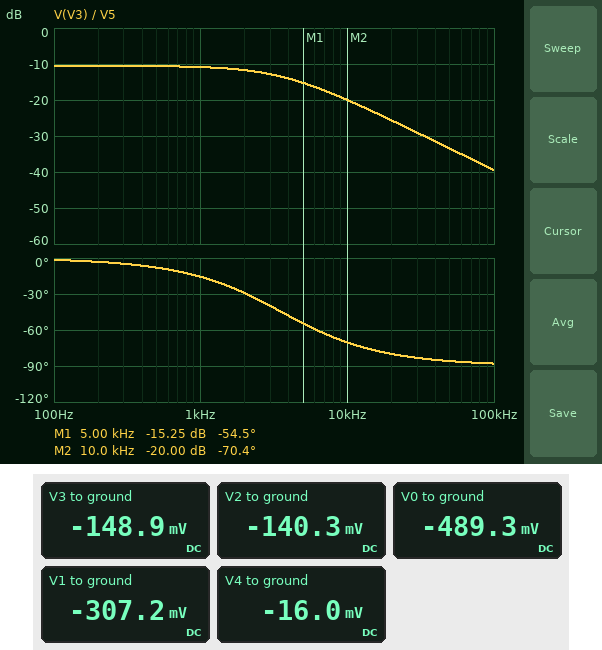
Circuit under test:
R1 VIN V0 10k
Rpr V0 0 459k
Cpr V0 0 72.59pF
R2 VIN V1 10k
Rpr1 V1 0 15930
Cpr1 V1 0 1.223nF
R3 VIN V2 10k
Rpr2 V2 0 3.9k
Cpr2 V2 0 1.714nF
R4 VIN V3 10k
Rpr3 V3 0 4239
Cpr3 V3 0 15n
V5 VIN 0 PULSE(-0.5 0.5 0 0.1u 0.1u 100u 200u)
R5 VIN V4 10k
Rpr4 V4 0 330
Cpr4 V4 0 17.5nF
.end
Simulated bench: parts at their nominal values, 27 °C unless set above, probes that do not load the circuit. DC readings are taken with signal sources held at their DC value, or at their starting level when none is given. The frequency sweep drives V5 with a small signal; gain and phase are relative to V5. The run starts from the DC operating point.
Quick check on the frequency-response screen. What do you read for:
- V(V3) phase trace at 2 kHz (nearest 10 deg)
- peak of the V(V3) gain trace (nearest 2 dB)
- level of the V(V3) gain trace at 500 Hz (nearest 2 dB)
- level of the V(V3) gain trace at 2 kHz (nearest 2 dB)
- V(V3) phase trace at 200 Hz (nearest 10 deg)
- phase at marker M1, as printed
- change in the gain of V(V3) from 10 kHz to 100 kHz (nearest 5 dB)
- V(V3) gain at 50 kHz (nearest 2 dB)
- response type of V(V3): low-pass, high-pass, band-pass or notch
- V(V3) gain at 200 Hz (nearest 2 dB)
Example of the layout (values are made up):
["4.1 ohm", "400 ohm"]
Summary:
["-30 deg", "-10 dB", "-10 dB", "-12 dB", "0 deg", "-54.5 deg", "-20 dB", "-34 dB", "low-pass", "-10 dB"]
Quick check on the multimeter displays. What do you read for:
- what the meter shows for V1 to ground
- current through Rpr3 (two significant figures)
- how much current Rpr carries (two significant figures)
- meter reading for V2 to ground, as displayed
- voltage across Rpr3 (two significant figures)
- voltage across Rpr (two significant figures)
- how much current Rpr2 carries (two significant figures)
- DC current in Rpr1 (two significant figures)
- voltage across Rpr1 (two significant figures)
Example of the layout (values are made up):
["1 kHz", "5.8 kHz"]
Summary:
["-307.2 mV", "35 µA", "1.1 µA", "-140.3 mV", "150 mV", "490 mV", "36 µA", "19 µA", "310 mV"]
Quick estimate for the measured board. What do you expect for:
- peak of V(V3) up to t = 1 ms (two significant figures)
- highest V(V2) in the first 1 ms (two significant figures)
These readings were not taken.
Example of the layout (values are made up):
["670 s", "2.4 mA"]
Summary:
["120 mV", "140 mV"]
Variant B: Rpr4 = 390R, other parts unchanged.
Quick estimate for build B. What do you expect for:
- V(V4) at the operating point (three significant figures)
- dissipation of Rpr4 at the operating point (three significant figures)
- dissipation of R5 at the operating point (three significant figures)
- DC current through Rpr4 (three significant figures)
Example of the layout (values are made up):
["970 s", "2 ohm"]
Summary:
["-18.8 mV", "903 nW", "23.2 µW", "48.1 µA"]
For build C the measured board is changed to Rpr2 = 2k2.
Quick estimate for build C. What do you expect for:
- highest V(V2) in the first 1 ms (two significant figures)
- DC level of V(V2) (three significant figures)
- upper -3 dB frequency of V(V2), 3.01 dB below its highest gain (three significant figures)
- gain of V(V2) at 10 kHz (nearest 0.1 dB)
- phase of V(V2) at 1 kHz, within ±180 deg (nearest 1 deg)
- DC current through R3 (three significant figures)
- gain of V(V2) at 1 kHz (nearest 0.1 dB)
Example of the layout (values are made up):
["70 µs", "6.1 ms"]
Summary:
["90 mV", "-90.2 mV", "51.5 kHz", "-15.0 dB", "-1 deg", "41.0 µA", "-14.9 dB"]
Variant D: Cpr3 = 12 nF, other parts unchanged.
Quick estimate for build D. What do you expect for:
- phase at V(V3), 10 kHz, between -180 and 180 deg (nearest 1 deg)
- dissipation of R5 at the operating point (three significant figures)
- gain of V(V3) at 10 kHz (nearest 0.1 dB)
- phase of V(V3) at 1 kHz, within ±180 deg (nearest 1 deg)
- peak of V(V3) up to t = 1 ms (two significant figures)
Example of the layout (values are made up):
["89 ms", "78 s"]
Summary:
["-66 deg", "23.4 µW", "-18.3 dB", "-13 deg", "130 mV"]
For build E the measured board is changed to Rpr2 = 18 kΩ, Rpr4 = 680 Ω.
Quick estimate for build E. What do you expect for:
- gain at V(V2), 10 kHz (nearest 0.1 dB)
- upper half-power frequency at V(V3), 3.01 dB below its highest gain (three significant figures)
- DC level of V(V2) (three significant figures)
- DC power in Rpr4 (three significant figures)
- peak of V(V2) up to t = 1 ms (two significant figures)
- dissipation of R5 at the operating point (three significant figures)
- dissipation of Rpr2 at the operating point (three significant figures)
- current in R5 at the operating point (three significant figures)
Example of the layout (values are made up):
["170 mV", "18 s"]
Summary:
["-5.5 dB", "3.56 kHz", "-321 mV", "1.49 µW", "320 mV", "21.9 µW", "5.74 µW", "46.8 µA"]
